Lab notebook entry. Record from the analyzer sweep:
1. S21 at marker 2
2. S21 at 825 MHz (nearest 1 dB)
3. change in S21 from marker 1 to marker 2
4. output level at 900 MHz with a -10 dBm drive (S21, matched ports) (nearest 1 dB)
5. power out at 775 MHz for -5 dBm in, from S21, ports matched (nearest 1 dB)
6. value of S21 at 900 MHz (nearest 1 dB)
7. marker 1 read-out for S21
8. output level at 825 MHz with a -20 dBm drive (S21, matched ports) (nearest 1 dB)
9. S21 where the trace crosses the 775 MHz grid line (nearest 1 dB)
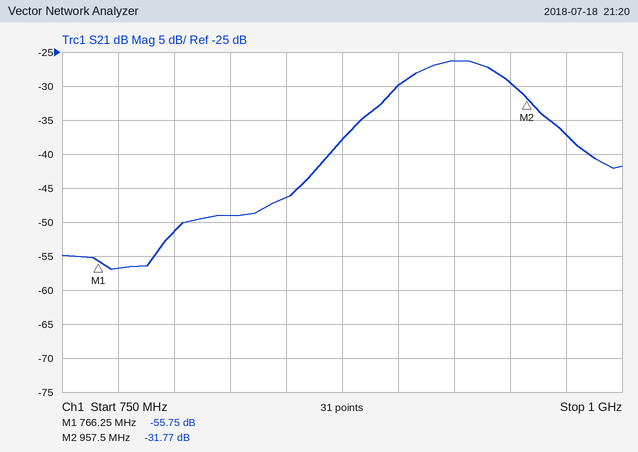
-31.77 dB
-49 dB
23.98 dB
-40 dBm
-62 dBm
-30 dB
-55.75 dB
-69 dBm
-57 dB
